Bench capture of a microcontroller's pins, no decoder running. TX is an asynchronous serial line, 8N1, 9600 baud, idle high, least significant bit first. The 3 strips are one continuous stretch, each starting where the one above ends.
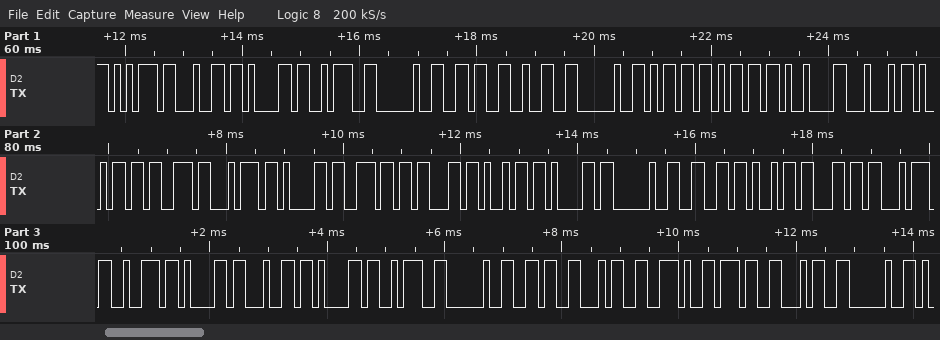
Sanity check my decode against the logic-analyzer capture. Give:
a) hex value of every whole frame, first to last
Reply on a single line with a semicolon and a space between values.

0x75 0x64 0x61 0x3A 0x20 0x36 0x32 0x20 0x6D 0x6D 0x09 0x44 0x69 0x73 0x74 0x61 0x6E 0x63 0x69 0x61 0x20 0x66 0x69 0x6C 0x74 0x72 0x61 0x64 0x61 0x3A 0x20 0x36 0x34 0x2E 0x37 0x34 0x20
